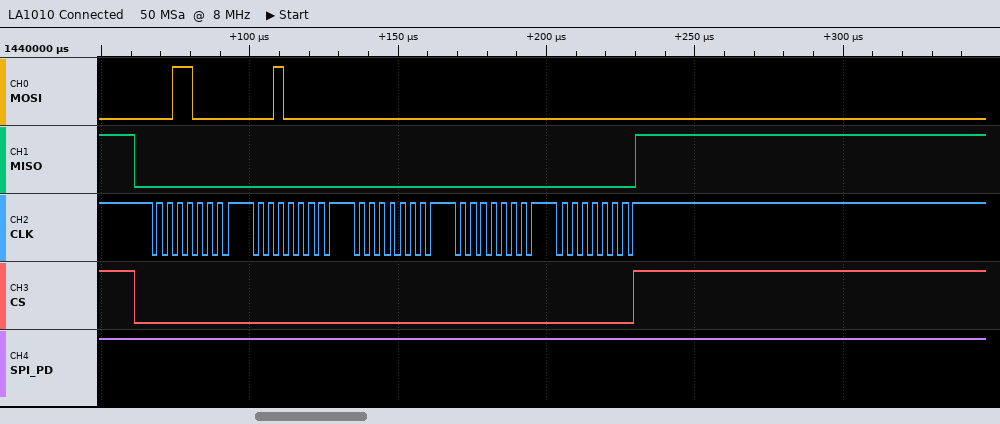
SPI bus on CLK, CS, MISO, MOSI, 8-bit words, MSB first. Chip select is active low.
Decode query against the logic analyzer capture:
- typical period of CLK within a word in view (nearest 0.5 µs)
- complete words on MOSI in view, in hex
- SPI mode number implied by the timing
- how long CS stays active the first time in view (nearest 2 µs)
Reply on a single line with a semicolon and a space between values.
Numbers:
3.5 µs; 30, 20, 00, 00, 00; 3; 168 µs
